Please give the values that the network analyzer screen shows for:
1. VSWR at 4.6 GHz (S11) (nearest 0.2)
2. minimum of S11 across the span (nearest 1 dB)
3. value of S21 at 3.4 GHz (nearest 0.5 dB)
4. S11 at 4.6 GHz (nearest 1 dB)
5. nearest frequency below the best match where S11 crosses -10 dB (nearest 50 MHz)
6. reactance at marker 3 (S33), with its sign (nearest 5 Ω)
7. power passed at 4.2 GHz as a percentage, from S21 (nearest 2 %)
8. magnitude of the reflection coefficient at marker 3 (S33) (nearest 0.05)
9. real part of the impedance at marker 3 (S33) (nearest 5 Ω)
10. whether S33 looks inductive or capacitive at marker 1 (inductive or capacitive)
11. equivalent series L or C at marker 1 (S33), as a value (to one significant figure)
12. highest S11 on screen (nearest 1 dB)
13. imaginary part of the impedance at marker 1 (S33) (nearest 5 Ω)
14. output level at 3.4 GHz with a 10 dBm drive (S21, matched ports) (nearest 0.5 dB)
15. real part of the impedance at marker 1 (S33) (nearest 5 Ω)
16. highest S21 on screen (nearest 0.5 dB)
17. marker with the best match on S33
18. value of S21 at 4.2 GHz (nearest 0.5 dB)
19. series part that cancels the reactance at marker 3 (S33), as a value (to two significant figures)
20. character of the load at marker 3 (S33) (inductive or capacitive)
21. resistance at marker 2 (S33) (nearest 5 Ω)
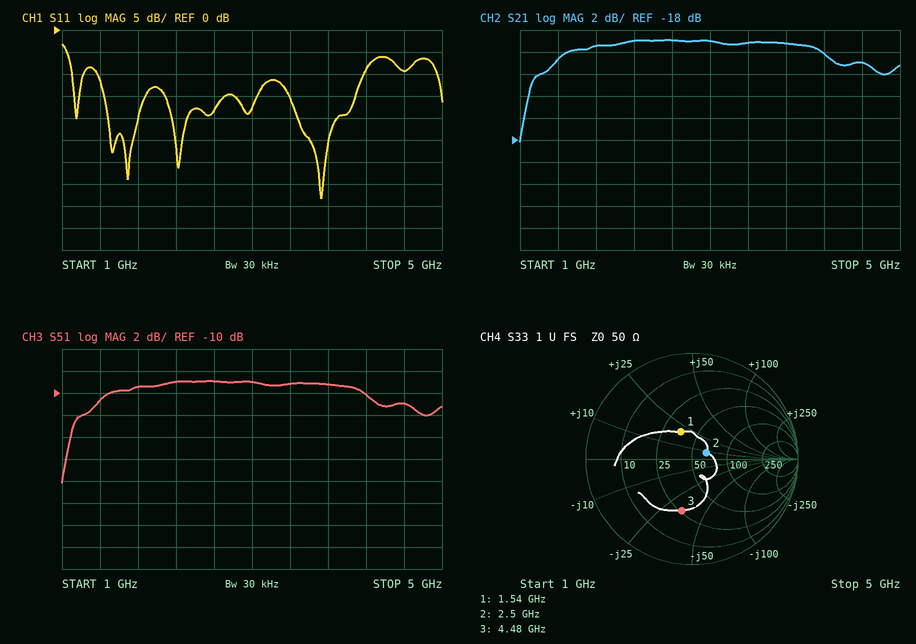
2.0
-38 dB
-9.0 dB
-9 dB
1.35 GHz
-35 Ω
10 %
0.50
25 Ω
inductive
2 nH
-3 dB
+20 Ω
1.0 dBm
35 Ω
-9.0 dB
marker 2
-10.0 dB
1.2 nH
capacitive
65 Ω
